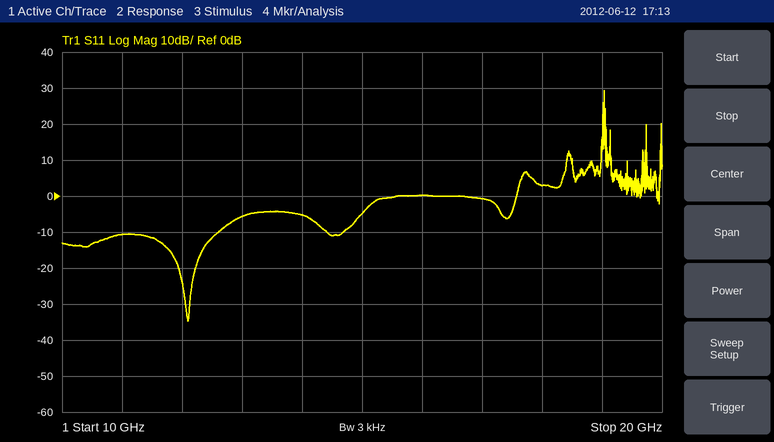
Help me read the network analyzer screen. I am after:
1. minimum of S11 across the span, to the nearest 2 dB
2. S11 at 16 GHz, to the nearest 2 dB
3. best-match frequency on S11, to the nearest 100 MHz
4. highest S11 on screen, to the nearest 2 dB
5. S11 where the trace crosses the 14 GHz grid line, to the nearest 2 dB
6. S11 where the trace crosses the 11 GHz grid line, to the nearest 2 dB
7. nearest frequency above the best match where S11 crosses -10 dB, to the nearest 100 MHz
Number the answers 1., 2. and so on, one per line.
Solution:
1. -34 dB
2. 0 dB
3. 12.1 GHz
4. 30 dB
5. -6 dB
6. -10 dB
7. 12.6 GHz
